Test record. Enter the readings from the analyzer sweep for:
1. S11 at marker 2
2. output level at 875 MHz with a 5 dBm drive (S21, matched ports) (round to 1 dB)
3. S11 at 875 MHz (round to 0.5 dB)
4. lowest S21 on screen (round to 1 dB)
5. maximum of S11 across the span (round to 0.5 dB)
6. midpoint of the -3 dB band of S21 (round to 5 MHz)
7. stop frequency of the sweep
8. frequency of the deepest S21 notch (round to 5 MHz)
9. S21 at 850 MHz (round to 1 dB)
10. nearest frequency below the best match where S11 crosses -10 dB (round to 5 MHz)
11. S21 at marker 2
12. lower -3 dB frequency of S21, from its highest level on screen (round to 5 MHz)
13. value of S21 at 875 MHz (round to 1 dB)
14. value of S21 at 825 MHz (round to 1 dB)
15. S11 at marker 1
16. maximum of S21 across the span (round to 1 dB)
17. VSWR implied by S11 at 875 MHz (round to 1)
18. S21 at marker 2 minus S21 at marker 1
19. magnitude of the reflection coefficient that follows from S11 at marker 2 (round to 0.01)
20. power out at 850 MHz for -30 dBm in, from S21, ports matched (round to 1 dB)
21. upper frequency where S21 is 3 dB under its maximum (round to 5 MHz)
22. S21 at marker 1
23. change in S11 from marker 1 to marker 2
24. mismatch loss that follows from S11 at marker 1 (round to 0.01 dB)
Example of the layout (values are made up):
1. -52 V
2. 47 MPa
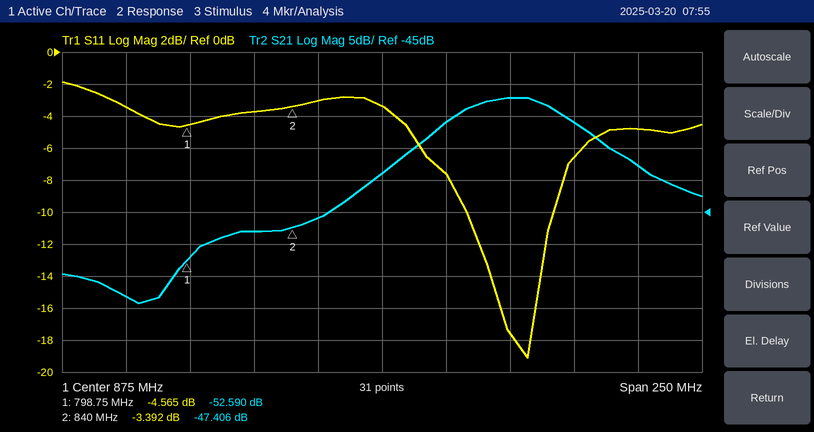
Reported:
1. -3.392 dB
2. -34 dBm
3. -3.5 dB
4. -59 dB
5. -2.0 dB
6. 925 MHz
7. 1 GHz
8. 780 MHz
9. -46 dB
10. 910 MHz
11. -47.406 dB
12. 905 MHz
13. -39 dB
14. -48 dB
15. -4.565 dB
16. -27 dB
17. 5
18. 5.184 dB
19. 0.68
20. -76 dBm
21. 945 MHz
22. -52.590 dB
23. 1.173 dB
24. 1.87 dB
